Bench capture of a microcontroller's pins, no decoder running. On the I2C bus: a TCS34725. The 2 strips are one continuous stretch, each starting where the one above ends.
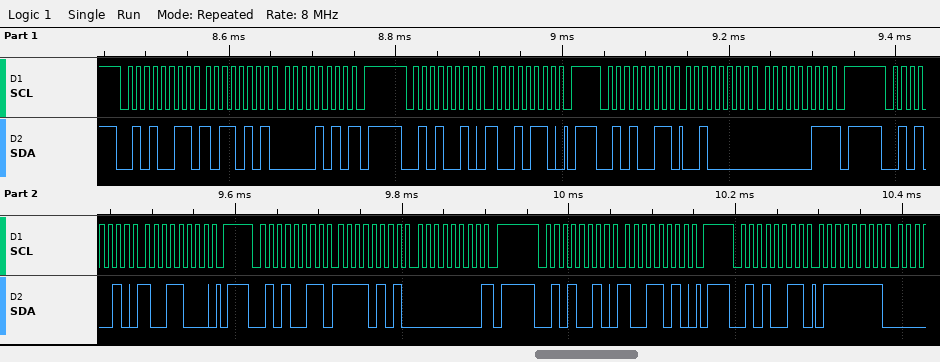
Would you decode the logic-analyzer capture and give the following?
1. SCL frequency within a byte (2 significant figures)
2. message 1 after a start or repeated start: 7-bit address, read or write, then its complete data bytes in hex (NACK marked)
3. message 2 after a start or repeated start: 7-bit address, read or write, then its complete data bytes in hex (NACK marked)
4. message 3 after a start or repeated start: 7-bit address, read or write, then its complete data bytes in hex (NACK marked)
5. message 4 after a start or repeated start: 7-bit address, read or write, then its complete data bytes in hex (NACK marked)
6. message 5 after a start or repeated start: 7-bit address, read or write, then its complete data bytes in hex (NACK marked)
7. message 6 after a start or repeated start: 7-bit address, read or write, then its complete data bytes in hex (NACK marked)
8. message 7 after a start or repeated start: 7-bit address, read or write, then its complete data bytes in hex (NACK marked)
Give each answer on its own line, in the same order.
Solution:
100 kHz
0x29 read: B5 0A NACK
0x29 write: 96
0x29 read: 20 03 NACK
0x29 write: 98
0x29 read: F5 00 NACK
0x29 write: 9A
0x29 read: 7F
